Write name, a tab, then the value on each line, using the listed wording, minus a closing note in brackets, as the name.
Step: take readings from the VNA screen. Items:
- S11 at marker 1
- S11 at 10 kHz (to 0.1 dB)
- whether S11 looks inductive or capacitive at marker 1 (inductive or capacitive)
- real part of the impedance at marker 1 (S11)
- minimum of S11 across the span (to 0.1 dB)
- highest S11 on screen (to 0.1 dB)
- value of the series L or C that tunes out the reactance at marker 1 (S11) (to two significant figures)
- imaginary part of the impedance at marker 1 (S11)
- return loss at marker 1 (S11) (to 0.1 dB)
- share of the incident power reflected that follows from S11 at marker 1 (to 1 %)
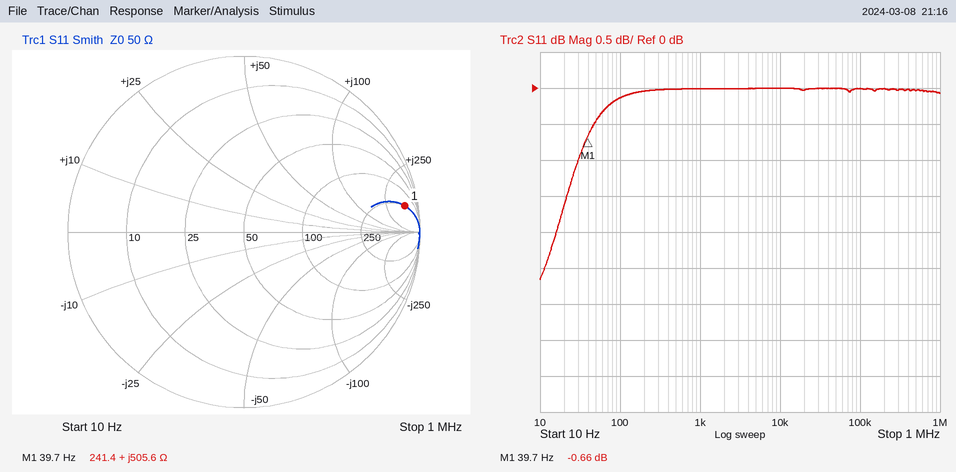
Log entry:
S11 at marker 1	-0.66 dB
S11 at 10 kHz	0.0 dB
whether S11 looks inductive or capacitive at marker 1	inductive
real part of the impedance at marker 1	241.4 Ω
minimum of S11 across the span	-2.7 dB
highest S11 on screen	0.0 dB
value of the series L or C that tunes out the reactance at marker 1 (S11)	7.9 µF
imaginary part of the impedance at marker 1	+505.6 Ω
return loss at marker 1 (S11)	0.7 dB
share of the incident power reflected that follows from S11 at marker 1	86 %
